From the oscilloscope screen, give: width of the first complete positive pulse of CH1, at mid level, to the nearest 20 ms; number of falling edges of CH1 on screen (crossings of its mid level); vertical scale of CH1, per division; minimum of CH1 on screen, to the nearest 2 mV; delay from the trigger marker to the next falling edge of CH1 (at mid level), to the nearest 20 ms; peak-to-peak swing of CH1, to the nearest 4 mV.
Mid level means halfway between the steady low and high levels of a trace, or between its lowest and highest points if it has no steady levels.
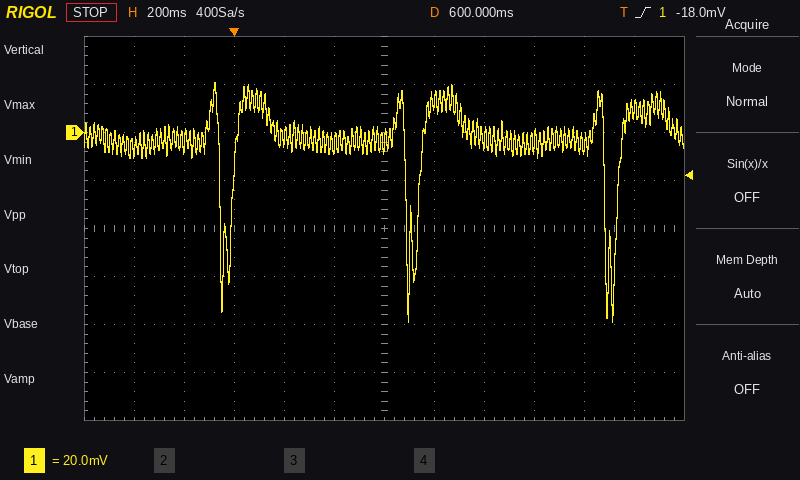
700 ms
3
20 mV
-78 mV
680 ms
100 mV
